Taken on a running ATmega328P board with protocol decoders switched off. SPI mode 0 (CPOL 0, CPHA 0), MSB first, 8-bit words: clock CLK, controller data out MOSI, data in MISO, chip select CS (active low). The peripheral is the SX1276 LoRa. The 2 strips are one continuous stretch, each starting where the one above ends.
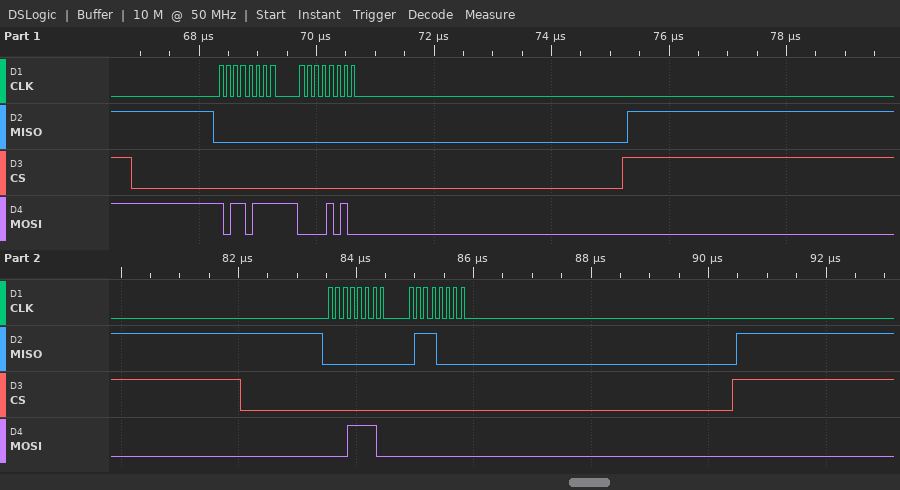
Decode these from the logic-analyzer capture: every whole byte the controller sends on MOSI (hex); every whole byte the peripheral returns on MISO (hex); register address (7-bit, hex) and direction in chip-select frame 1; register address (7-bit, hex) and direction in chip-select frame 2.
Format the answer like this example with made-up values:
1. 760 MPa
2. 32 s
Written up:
1. B7 0A 1E 00
2. 00 00 00 70
3. 0x37 write
4. 0x1E read
